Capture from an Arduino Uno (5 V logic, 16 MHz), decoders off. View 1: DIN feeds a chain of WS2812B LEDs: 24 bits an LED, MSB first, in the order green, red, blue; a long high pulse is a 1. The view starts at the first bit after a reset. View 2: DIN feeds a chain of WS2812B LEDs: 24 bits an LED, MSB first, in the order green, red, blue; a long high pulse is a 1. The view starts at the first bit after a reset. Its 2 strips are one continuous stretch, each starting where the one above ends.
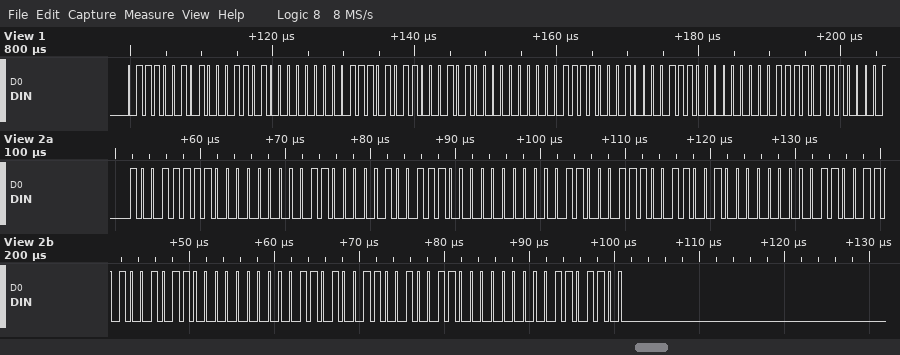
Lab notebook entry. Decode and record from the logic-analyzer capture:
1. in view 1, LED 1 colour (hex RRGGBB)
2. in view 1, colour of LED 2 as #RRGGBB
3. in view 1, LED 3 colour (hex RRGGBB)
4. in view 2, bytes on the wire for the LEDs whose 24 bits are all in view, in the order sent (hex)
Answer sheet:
#8D7200
#8A7500
#877800
9F 00 60 9C 00 63 99 00 66 96 00 69 93 00 6C
